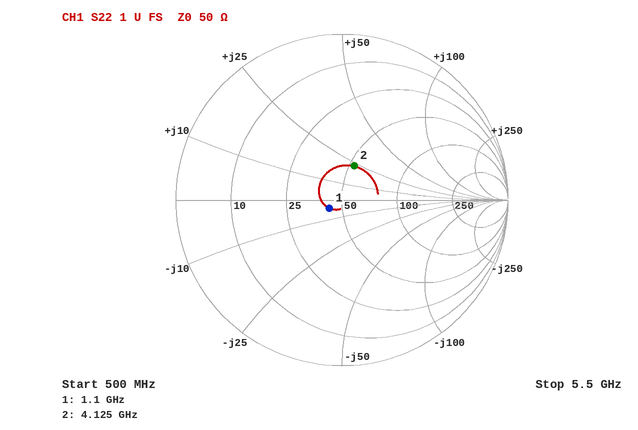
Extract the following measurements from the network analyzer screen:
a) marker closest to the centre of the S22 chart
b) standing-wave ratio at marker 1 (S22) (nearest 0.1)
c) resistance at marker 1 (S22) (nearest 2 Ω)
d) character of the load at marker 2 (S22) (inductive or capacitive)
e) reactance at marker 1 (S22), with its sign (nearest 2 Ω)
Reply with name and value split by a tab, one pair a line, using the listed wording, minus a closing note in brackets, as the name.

marker closest to the centre of the S22 chart	marker 1
standing-wave ratio at marker 1 (S22)	1.2
resistance at marker 1 (S22)	42 Ω
character of the load at marker 2 (S22)	inductive
reactance at marker 1 (S22), with its sign	-4 Ω
